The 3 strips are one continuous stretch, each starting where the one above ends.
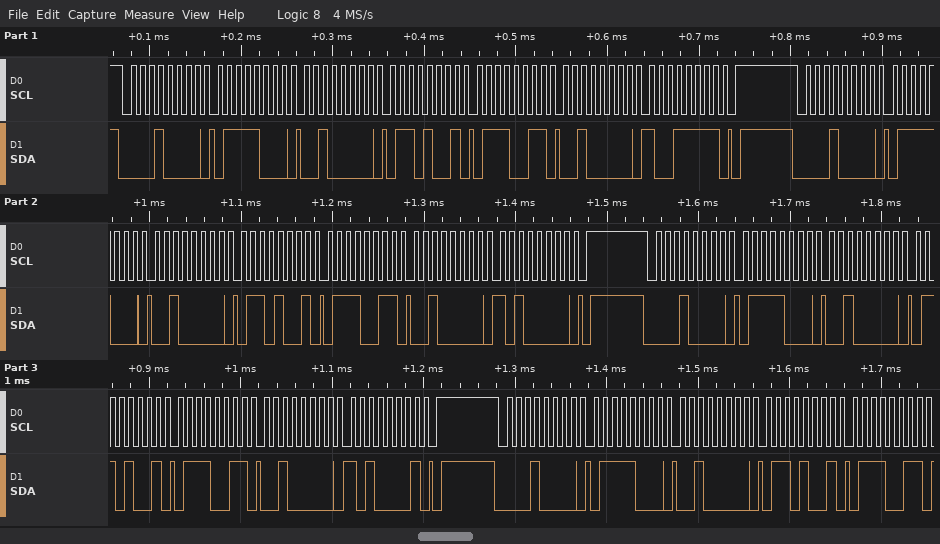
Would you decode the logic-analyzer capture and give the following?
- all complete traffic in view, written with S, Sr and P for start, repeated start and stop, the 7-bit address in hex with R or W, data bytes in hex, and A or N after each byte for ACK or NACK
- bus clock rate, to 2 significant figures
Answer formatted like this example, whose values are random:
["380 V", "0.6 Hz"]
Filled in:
["S 08W A 78 A 20 A 69 A 73 A 20 A 9F A P S 08W A 78 A 20 A 69 A 73 A 20 A A0 A P S 08W A 78 A 20 A 69 A 73 A 20 A A1 A P S 08W A 78 A 20 A 69 A 73 A", "100 kHz"]
